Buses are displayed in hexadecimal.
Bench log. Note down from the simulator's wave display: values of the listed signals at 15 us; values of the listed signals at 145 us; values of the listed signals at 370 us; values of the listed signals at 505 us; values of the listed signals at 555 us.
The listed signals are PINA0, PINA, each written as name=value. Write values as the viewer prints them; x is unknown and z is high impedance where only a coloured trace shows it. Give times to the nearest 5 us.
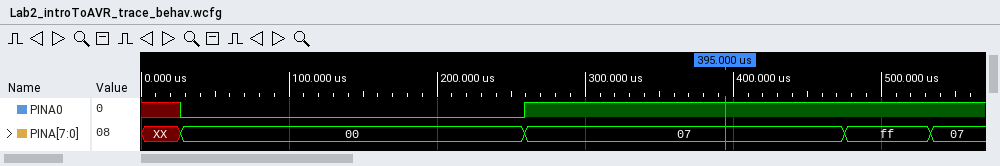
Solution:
PINA0=x, PINA=XX
PINA0=0, PINA=00
PINA0=1, PINA=07
PINA0=1, PINA=ff
PINA0=1, PINA=07
